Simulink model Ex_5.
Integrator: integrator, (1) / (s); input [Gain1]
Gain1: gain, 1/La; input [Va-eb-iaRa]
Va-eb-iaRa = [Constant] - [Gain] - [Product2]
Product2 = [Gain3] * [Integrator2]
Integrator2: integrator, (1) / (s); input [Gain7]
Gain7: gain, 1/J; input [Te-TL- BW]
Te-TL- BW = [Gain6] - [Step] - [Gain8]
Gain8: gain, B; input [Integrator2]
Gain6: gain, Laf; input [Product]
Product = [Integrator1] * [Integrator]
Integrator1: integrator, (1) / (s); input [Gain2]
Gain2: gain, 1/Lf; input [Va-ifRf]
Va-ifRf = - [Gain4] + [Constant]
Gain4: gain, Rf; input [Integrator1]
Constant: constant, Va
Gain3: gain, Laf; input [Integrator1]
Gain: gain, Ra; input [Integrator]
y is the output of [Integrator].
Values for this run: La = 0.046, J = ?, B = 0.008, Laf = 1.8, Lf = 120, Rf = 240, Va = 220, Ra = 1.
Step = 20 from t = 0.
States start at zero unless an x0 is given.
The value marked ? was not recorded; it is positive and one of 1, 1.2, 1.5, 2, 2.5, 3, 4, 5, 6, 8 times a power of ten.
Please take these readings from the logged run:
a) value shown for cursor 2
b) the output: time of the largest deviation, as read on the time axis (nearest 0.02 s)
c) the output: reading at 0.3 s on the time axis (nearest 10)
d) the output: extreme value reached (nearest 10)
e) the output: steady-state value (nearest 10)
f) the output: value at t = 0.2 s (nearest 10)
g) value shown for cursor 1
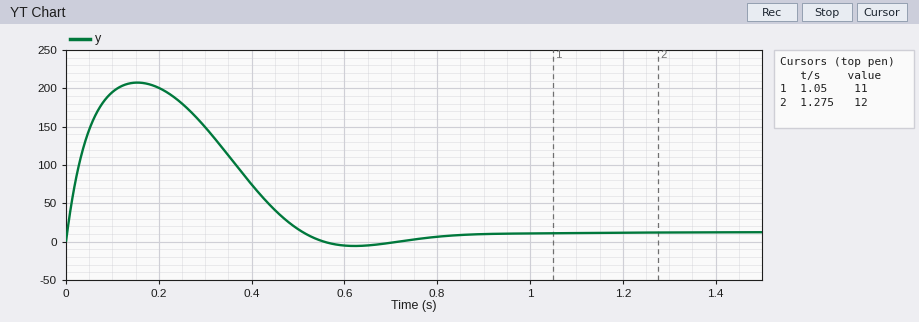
12
0.16 s
150
210
10
200
11
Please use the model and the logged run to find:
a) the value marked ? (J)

0.12
